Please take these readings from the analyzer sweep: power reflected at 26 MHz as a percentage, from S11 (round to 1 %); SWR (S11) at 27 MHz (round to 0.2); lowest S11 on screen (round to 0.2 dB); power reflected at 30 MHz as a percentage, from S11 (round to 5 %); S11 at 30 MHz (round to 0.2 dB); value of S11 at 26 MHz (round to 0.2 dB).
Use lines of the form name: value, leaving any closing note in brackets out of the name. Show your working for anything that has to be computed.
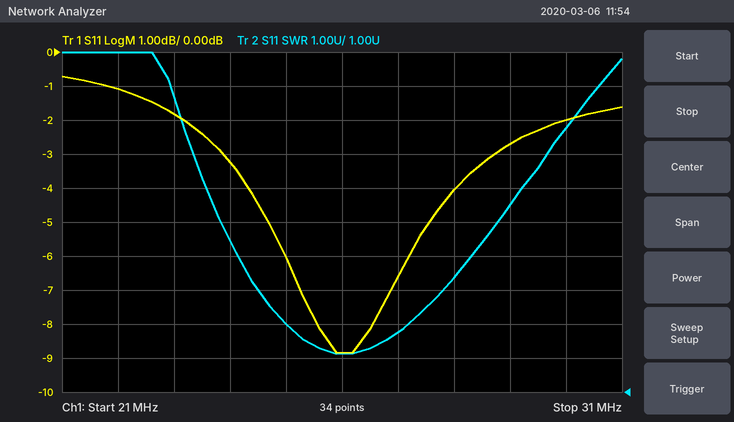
power reflected at 26 MHz as a percentage, from S11: 10^(-8.8/10) ≈ 13 %
SWR (S11) at 27 MHz: 2.8
lowest S11 on screen: -8.8 dB
power reflected at 30 MHz as a percentage, from S11: 10^(-2/10) ≈ 63.1 %, so 65 % to the nearest 5 %
S11 at 30 MHz: -2.0 dB
value of S11 at 26 MHz: -8.8 dB
